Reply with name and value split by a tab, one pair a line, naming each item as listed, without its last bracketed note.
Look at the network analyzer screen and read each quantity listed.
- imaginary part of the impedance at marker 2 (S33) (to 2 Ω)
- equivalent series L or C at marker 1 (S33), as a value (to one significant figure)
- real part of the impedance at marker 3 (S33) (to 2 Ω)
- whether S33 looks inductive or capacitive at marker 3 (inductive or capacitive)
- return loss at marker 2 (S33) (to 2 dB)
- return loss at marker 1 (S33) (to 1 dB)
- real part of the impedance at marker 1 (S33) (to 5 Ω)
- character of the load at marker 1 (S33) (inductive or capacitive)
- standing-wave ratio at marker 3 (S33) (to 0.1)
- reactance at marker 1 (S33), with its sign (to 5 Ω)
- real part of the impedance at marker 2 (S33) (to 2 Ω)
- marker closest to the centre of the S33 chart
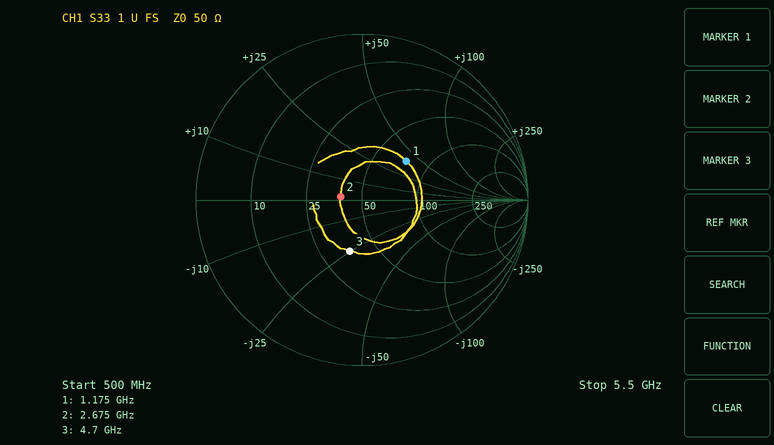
imaginary part of the impedance at marker 2 (S33)	+2 Ω
equivalent series L or C at marker 1 (S33), as a value	5 nH
real part of the impedance at marker 3 (S33)	36 Ω
whether S33 looks inductive or capacitive at marker 3	capacitive
return loss at marker 2 (S33)	18 dB
return loss at marker 1 (S33)	9 dB
real part of the impedance at marker 1 (S33)	75 Ω
character of the load at marker 1 (S33)	inductive
standing-wave ratio at marker 3 (S33)	1.9
reactance at marker 1 (S33), with its sign	+40 Ω
real part of the impedance at marker 2 (S33)	38 Ω
marker closest to the centre of the S33 chart	marker 2
